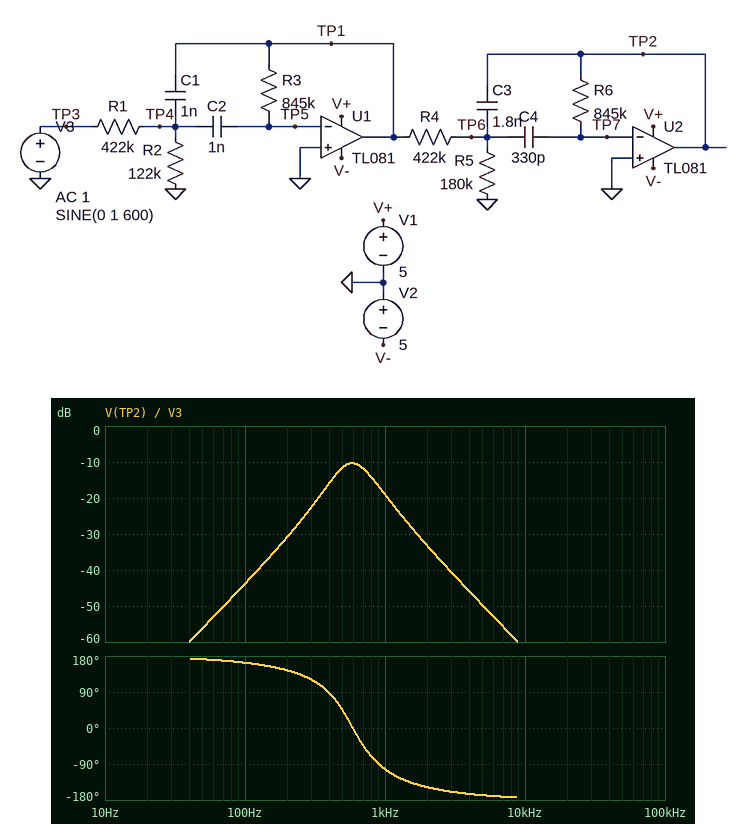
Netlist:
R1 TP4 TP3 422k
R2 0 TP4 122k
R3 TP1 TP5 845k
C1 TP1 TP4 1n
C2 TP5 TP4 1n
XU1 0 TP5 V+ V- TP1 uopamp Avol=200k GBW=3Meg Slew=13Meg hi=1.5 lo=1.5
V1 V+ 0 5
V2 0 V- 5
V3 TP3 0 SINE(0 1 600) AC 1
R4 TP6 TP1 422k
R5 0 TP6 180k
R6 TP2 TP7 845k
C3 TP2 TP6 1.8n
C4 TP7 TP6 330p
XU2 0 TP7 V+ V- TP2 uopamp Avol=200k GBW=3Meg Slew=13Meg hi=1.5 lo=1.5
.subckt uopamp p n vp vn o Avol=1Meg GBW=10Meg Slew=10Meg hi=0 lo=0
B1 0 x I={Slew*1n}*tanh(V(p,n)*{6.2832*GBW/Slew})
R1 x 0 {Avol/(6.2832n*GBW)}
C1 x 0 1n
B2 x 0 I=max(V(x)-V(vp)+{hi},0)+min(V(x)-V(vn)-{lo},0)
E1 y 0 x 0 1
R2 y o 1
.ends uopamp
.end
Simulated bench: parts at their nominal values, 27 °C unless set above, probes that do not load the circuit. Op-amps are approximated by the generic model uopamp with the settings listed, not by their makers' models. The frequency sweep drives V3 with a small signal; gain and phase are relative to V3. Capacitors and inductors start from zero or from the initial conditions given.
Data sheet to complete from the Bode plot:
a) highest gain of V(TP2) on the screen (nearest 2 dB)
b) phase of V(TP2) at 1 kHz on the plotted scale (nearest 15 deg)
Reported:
-10 dB
-105 deg
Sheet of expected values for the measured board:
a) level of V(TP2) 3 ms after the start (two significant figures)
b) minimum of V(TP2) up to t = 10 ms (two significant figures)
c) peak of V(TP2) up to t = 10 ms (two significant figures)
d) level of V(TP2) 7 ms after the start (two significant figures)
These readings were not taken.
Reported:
-280 mV
-300 mV
300 mV
280 mV
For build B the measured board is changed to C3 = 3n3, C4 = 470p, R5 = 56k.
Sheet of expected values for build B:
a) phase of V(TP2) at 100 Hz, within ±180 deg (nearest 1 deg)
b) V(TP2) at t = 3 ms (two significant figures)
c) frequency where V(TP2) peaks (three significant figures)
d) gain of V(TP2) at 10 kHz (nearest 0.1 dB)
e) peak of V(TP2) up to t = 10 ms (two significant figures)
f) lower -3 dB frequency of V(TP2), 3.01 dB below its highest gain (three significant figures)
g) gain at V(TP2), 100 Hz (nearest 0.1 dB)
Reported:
166 deg
-210 mV
590 Hz
-67.3 dB
240 mV
470 Hz
-48.8 dB
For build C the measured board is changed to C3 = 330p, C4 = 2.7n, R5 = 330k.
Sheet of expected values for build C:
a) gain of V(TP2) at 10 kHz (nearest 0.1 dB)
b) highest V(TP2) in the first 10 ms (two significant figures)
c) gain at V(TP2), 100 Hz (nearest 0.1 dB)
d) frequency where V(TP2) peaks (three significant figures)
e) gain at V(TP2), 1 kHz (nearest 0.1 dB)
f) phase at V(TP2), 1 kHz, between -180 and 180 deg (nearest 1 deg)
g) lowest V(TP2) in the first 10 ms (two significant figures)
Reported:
-47.3 dB
1.6 V
-22.4 dB
538 Hz
-5.5 dB
-113 deg
-1.6 V
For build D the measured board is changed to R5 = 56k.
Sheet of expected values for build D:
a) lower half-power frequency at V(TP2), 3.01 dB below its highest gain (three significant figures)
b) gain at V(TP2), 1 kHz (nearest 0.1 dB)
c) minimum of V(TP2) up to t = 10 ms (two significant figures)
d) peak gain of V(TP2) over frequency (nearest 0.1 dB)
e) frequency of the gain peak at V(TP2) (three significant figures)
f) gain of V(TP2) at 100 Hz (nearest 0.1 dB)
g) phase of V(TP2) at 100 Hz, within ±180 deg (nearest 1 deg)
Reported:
510 Hz
-16.5 dB
-160 mV
-15.2 dB
755 Hz
-52.0 dB
169 deg
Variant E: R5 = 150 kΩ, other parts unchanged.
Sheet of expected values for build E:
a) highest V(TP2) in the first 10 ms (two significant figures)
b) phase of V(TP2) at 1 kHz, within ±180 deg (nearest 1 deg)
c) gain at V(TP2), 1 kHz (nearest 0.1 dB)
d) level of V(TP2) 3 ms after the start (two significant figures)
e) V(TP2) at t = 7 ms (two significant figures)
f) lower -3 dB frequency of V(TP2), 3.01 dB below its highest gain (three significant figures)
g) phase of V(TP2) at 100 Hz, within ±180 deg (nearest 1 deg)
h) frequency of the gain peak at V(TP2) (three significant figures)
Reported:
300 mV
-100 deg
-18.7 dB
-260 mV
290 mV
461 Hz
164 deg
595 Hz
